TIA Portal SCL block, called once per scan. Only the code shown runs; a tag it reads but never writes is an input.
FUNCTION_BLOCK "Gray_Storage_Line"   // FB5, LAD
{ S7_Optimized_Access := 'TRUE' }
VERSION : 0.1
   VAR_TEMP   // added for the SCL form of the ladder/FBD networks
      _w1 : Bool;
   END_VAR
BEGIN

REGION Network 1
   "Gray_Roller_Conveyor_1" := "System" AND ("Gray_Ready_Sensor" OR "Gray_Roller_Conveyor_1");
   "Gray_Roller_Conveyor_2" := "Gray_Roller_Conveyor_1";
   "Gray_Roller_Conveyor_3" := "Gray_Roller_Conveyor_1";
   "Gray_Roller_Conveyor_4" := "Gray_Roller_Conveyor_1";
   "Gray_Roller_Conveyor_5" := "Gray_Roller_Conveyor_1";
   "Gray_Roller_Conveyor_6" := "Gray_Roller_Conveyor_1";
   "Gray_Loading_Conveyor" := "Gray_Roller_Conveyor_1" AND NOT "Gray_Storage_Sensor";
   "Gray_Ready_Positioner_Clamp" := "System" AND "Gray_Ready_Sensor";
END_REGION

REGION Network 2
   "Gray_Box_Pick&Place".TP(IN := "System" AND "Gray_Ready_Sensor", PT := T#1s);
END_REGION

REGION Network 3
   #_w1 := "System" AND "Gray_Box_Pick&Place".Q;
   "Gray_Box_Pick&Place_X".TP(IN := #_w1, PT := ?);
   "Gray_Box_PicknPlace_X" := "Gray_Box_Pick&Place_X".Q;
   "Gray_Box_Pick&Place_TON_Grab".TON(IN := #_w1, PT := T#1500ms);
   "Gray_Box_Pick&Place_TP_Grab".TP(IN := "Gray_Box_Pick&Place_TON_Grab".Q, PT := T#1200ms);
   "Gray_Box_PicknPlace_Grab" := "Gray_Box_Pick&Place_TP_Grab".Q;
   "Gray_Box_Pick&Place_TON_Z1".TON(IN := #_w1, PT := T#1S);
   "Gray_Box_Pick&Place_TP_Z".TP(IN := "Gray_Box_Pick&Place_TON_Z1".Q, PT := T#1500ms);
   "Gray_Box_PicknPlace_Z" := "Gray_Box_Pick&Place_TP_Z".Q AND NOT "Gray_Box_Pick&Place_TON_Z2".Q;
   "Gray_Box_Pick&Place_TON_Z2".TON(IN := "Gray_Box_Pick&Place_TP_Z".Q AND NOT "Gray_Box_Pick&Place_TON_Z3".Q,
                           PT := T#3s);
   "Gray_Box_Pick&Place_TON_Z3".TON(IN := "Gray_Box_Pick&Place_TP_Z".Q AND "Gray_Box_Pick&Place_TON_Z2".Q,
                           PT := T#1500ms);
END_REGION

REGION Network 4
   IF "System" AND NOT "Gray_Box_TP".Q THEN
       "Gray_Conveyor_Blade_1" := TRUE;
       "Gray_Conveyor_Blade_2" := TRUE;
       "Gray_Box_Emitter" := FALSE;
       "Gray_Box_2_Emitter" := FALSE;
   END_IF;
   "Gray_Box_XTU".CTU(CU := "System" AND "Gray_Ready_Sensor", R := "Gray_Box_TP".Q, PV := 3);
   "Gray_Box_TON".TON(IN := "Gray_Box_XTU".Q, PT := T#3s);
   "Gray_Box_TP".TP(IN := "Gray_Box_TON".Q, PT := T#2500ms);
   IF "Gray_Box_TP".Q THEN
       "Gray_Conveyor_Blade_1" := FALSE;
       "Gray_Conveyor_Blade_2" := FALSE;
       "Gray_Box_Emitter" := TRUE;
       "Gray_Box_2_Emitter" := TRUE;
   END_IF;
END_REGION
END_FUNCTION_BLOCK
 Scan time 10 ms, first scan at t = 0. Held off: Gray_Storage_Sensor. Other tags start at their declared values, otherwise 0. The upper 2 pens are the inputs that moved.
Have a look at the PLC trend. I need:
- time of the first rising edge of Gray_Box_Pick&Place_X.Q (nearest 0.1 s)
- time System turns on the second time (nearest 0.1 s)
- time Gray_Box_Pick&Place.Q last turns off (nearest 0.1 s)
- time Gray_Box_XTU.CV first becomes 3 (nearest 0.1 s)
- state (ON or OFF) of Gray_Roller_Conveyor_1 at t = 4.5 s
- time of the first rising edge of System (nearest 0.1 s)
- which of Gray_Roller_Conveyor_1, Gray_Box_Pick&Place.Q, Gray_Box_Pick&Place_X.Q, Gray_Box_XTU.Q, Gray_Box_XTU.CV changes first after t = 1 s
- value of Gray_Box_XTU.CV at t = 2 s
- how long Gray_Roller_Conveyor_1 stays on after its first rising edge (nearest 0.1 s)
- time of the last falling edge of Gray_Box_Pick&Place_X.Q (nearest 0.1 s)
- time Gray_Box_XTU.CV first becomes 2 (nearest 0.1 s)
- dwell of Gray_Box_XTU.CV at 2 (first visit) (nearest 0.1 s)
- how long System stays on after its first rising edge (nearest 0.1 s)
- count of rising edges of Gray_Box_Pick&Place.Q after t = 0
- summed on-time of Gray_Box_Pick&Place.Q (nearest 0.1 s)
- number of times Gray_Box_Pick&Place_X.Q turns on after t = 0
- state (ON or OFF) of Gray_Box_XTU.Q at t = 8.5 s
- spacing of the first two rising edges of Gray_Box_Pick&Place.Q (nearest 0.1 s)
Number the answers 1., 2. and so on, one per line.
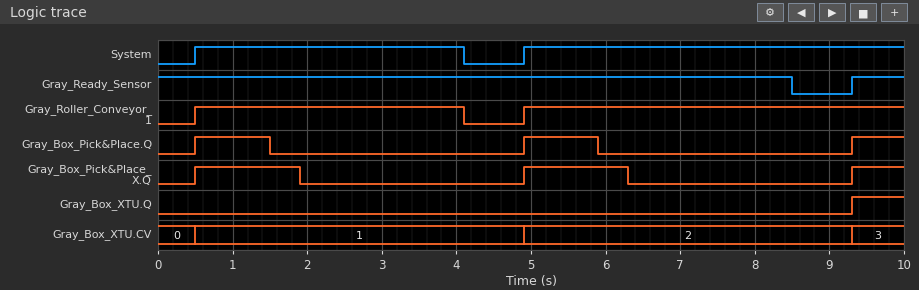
1. 0.5 s
2. 4.9 s
3. 5.9 s
4. 9.3 s
5. OFF
6. 0.5 s
7. Gray_Box_Pick&Place.Q
8. 1
9. 3.6 s
10. 6.3 s
11. 4.9 s
12. 4.4 s
13. 3.6 s
14. 3
15. 2.7 s
16. 3
17. OFF
18. 4.4 s
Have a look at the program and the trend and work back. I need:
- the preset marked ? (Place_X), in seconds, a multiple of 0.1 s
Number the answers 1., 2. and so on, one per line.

1. 1.4 s
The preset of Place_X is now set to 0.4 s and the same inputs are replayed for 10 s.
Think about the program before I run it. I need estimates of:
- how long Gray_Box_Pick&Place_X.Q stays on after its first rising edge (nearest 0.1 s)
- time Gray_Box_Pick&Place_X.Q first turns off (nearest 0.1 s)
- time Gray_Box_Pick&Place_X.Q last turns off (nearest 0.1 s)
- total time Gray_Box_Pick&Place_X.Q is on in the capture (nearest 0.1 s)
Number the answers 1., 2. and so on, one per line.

1. 0.4 s
2. 0.9 s
3. 9.7 s
4. 1.2 s
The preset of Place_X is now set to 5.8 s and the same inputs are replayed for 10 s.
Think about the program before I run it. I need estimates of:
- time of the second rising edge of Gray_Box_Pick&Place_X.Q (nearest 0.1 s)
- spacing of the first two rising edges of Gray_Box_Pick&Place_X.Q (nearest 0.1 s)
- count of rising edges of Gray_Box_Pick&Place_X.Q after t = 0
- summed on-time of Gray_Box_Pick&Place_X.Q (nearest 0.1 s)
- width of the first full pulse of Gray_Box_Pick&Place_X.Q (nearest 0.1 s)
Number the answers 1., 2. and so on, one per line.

1. 9.3 s
2. 8.8 s
3. 2
4. 6.5 s
5. 5.8 s
